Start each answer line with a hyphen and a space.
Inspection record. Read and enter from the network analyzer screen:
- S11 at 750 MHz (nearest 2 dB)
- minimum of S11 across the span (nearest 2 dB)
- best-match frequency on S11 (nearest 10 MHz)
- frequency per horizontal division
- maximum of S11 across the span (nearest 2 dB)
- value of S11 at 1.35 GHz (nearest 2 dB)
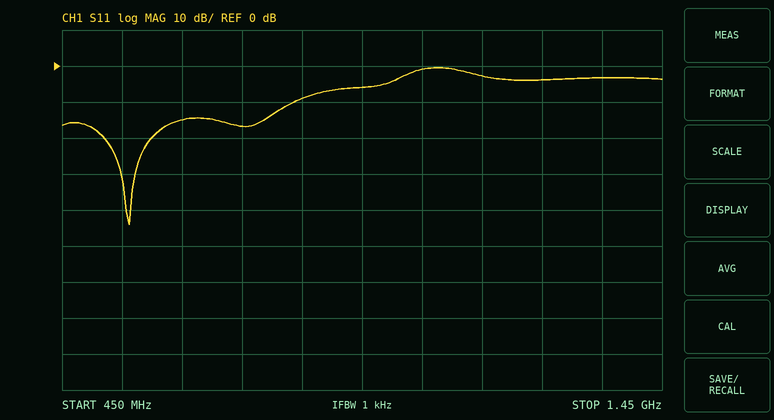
- -16 dB
- -44 dB
- 560 MHz
- 100 MHz
- 0 dB
- -4 dB
